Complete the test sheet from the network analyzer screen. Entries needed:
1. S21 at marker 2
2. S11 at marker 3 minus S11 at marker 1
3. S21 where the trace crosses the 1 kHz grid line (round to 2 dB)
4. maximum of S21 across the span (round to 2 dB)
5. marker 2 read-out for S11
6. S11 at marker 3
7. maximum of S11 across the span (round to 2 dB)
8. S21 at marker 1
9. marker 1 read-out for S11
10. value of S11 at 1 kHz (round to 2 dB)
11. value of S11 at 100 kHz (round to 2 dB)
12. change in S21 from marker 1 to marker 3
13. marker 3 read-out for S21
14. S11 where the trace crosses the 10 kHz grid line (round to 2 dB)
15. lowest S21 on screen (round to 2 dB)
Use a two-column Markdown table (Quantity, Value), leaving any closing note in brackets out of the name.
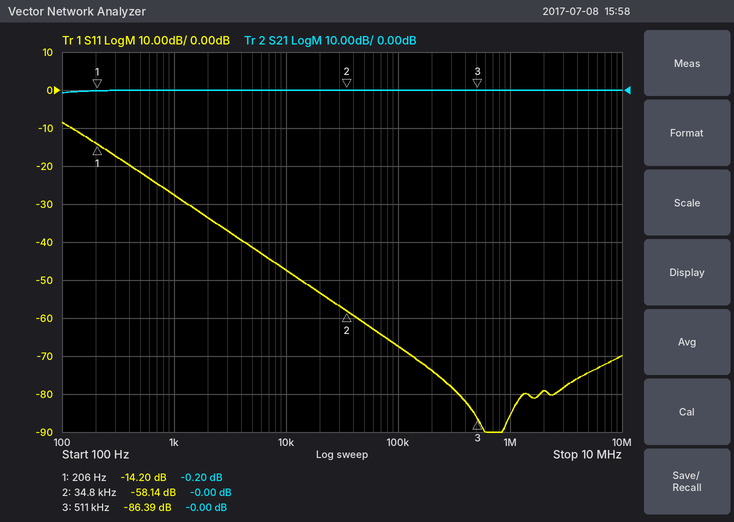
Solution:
| Quantity | Value |
|---|---|
| S21 at marker 2 | -0.00 dB |
| S11 at marker 3 minus S11 at marker 1 | -72.19 dB |
| S21 where the trace crosses the 1 kHz grid line | 0 dB |
| maximum of S21 across the span | 0 dB |
| marker 2 read-out for S11 | -58.14 dB |
| S11 at marker 3 | -86.39 dB |
| maximum of S11 across the span | -8 dB |
| S21 at marker 1 | -0.20 dB |
| marker 1 read-out for S11 | -14.20 dB |
| value of S11 at 1 kHz | -28 dB |
| value of S11 at 100 kHz | -68 dB |
| change in S21 from marker 1 to marker 3 | 0.20 dB |
| marker 3 read-out for S21 | -0.00 dB |
| S11 where the trace crosses the 10 kHz grid line | -48 dB |
| lowest S21 on screen | 0 dB |
